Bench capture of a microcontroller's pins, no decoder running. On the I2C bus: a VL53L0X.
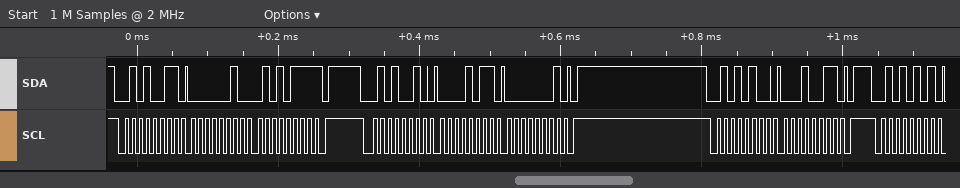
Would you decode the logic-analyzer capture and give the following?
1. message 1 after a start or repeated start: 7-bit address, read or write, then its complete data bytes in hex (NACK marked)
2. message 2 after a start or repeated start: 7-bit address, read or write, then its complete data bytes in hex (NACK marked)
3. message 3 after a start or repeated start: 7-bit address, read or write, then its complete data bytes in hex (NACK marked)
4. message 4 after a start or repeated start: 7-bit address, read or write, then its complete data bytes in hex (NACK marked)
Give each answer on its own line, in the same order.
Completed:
0x29 read: 02 57 NACK
0x29 write: 0B 01
0x2A write: 13
0x2A read
